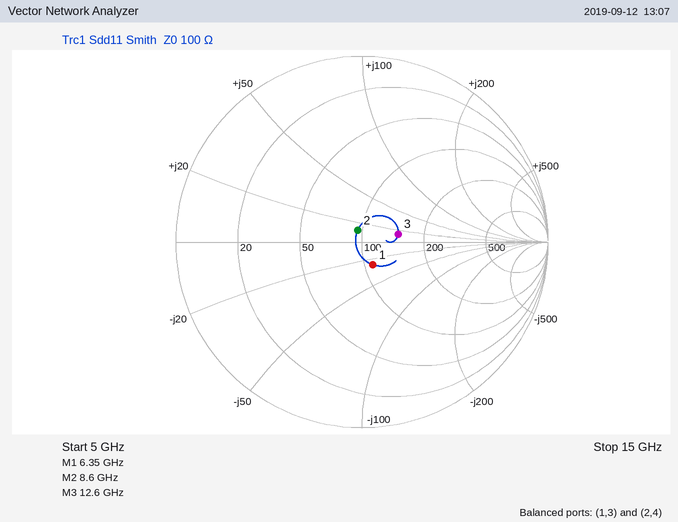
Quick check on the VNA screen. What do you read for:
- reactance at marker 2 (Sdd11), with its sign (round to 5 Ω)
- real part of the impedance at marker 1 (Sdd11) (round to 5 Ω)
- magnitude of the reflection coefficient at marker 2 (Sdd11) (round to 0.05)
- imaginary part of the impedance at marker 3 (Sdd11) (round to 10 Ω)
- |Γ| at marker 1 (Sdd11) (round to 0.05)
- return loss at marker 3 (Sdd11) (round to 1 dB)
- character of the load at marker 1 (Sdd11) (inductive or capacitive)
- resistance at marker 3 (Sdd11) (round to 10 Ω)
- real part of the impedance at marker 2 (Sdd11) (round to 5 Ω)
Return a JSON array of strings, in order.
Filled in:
["+10 Ω", "110 Ω", "0.05", "+10 Ω", "0.15", "14 dB", "capacitive", "150 Ω", "95 Ω"]
